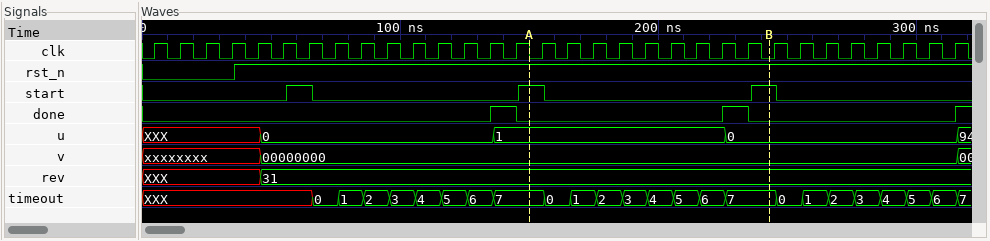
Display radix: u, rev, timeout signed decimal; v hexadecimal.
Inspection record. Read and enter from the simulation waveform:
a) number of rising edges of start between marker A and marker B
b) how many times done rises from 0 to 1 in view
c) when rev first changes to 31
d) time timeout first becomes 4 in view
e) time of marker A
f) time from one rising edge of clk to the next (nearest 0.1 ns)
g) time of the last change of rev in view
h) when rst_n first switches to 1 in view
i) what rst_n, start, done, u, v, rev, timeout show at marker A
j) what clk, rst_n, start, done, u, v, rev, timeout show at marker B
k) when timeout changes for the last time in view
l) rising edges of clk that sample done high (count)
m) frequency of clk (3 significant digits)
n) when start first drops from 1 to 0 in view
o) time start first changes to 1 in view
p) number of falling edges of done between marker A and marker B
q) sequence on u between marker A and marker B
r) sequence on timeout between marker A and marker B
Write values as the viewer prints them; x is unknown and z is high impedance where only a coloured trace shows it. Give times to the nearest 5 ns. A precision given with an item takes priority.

1
3
45 ns
105 ns
150 ns
10 ns
45 ns
35 ns
rst_n=1, start=1, done=0, u=1, v=00000000, rev=31, timeout=7
clk=0, rst_n=1, start=1, done=0, u=0, v=00000000, rev=31, timeout=7
315 ns
2
100 MHz
65 ns
55 ns
1
1, 0
7, 0, 1, 2, 3, 4, 5, 6, 7
